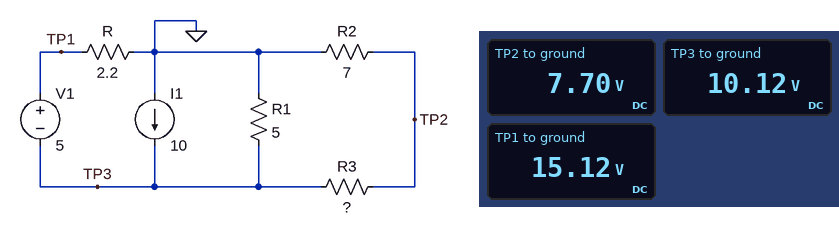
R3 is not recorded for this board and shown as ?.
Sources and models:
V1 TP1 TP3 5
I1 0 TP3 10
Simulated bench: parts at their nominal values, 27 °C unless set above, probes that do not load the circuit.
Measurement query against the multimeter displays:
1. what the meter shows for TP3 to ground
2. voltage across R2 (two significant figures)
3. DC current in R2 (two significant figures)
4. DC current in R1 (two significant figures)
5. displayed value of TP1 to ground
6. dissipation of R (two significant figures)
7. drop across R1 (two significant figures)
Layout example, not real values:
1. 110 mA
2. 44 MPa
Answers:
1. 10.12 V
2. 7.7 V
3. 1.1 A
4. 2.0 A
5. 15.12 V
6. 100 W
7. 10 V
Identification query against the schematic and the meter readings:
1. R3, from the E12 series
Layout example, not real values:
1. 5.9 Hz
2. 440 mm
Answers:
1. 2.2 Ω
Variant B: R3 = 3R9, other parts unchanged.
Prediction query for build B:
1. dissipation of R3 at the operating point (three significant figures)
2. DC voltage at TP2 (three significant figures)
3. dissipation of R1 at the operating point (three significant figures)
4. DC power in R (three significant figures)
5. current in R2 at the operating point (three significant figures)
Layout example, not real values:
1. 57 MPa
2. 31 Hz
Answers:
1. 3.52 W
2. 6.65 V
3. 21.4 W
4. 107 W
5. 950 mA
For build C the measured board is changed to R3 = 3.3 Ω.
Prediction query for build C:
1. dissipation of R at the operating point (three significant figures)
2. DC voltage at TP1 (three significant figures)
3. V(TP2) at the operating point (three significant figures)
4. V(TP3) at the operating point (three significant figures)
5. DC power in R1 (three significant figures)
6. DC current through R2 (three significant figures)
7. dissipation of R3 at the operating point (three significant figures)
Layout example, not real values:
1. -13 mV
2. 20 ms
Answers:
1. 106 W
2. 15.3 V
3. 6.99 V
4. 10.3 V
5. 21.1 W
6. 998 mA
7. 3.29 W
